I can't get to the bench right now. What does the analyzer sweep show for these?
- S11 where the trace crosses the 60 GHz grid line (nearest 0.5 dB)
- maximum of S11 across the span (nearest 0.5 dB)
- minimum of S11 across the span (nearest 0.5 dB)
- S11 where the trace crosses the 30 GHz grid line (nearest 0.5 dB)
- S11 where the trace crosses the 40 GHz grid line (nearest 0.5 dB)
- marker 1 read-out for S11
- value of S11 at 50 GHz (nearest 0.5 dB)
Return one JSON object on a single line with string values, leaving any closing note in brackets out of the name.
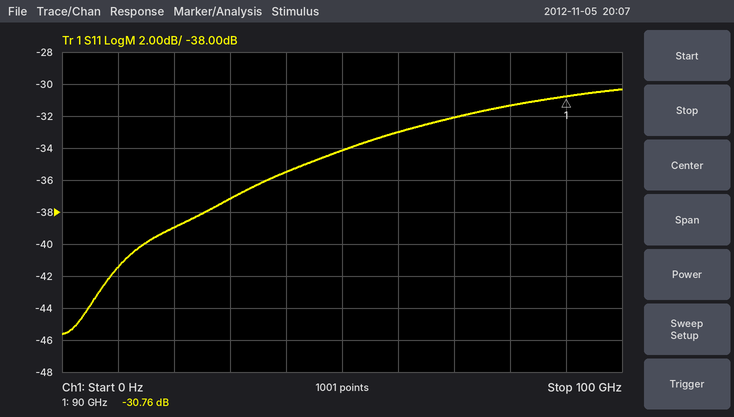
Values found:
{"S11 where the trace crosses the 60 GHz grid line": "-33.0 dB", "maximum of S11 across the span": "-30.5 dB", "minimum of S11 across the span": "-45.5 dB", "S11 where the trace crosses the 30 GHz grid line": "-37.0 dB", "S11 where the trace crosses the 40 GHz grid line": "-35.5 dB", "marker 1 read-out for S11": "-30.76 dB", "value of S11 at 50 GHz": "-34.0 dB"}
